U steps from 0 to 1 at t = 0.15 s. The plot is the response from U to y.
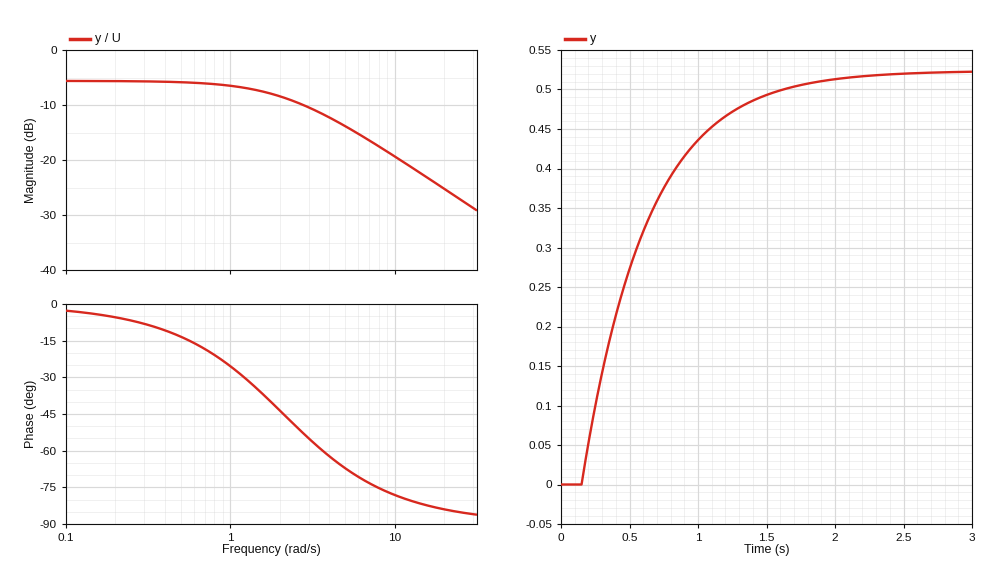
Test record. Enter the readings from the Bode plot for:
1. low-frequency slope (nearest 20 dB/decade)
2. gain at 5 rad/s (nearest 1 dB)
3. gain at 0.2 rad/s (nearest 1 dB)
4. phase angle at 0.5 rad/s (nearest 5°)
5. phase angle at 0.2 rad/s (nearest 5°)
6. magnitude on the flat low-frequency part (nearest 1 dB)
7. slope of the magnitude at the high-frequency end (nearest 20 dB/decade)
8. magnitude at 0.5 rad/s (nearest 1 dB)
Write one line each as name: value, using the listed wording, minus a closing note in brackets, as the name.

low-frequency slope: 0 dB/decade
gain at 5 rad/s: -14 dB
gain at 0.2 rad/s: -6 dB
phase angle at 0.5 rad/s: -15°
phase angle at 0.2 rad/s: -5°
magnitude on the flat low-frequency part: -6 dB
slope of the magnitude at the high-frequency end: -20 dB/decade
magnitude at 0.5 rad/s: -6 dB
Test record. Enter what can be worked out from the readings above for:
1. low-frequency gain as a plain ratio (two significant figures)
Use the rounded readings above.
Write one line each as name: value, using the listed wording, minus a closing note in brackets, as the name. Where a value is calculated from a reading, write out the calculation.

low-frequency gain as a plain ratio: 10^(-6 / 20) = 0.50
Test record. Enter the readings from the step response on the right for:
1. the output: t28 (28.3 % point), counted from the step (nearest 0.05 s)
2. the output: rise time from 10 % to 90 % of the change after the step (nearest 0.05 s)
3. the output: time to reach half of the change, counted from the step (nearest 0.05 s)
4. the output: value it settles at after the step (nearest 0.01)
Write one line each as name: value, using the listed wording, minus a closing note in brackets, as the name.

the output: t28 (28.3 % point), counted from the step: 0.15 s
the output: rise time from 10 % to 90 % of the change after the step: 1.05 s
the output: time to reach half of the change, counted from the step: 0.35 s
the output: value it settles at after the step: 0.52
